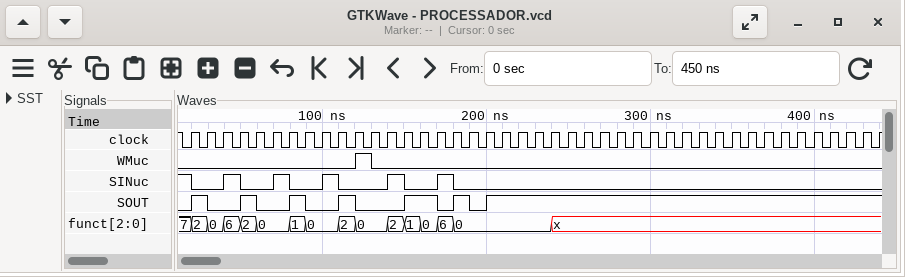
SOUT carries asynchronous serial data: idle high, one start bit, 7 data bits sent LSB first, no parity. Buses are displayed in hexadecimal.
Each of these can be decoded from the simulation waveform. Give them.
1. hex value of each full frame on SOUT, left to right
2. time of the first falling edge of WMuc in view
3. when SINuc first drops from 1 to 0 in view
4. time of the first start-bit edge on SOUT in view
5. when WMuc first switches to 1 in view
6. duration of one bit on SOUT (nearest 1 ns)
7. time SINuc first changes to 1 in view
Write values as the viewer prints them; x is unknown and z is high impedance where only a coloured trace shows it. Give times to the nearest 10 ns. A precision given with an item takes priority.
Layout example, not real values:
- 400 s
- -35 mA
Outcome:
- 12, 2C
- 130 ns
- 20 ns
- 30 ns
- 120 ns
- 10 ns
- 40 ns
